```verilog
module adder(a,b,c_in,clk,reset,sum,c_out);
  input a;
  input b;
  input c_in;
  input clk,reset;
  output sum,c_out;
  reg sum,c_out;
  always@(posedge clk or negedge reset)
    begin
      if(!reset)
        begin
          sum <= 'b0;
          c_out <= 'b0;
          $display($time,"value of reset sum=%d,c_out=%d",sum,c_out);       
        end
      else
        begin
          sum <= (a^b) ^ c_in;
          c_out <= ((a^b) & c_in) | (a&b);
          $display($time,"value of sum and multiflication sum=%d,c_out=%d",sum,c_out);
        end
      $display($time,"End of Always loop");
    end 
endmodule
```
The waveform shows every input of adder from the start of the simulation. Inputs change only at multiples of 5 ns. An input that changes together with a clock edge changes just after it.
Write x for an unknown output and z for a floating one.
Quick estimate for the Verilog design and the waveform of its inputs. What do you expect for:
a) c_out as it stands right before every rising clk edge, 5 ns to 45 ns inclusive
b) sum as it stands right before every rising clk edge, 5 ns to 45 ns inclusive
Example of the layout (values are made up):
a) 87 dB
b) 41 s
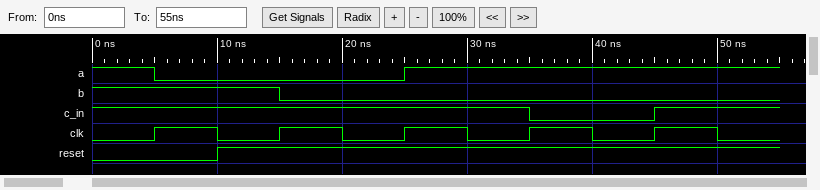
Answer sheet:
a) 0 0 1 0 1
b) 0 0 0 1 0
